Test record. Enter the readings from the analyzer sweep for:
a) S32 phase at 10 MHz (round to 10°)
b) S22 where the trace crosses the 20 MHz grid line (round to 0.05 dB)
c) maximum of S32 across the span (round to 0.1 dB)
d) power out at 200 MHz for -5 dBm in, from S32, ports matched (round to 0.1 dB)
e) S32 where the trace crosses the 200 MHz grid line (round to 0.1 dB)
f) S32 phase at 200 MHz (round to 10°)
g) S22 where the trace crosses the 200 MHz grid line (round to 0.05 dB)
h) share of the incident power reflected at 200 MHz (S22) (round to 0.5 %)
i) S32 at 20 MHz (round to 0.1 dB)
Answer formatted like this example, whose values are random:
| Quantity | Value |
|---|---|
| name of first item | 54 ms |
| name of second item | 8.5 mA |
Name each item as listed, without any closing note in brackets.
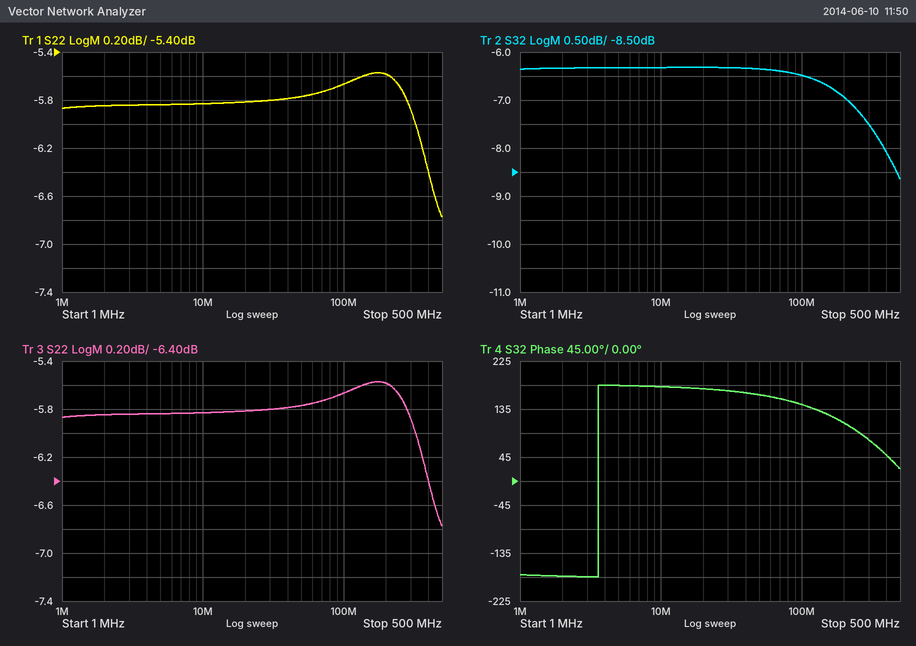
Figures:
| Quantity | Value |
|---|---|
| S32 phase at 10 MHz | 180° |
| S22 where the trace crosses the 20 MHz grid line | -5.80 dB |
| maximum of S32 across the span | -6.3 dB |
| power out at 200 MHz for -5 dBm in, from S32, ports matched | -11.9 dBm |
| S32 where the trace crosses the 200 MHz grid line | -6.9 dB |
| S32 phase at 200 MHz | 110° |
| S22 where the trace crosses the 200 MHz grid line | -5.60 dB |
| share of the incident power reflected at 200 MHz (S22) | 27.5 % |
| S32 at 20 MHz | -6.3 dB |
